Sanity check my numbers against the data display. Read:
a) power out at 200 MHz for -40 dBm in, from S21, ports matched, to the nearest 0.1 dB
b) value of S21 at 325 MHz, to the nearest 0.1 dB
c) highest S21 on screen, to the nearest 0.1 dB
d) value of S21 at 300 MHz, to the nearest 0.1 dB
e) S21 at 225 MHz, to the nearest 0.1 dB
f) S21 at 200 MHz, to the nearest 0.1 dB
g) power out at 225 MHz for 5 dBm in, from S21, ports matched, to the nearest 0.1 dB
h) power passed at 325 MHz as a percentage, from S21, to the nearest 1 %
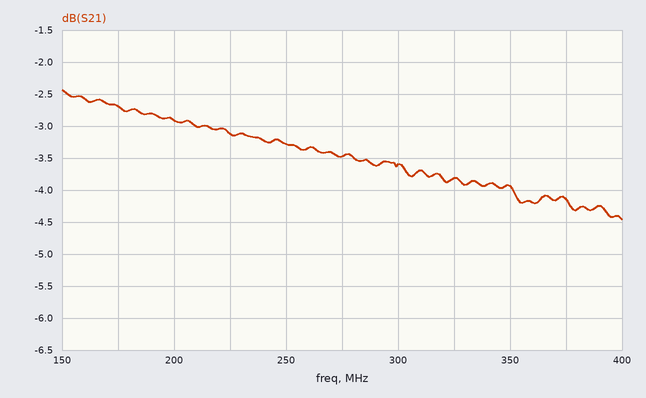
-42.9 dBm
-3.8 dB
-2.4 dB
-3.6 dB
-3.1 dB
-2.9 dB
1.9 dBm
42 %
